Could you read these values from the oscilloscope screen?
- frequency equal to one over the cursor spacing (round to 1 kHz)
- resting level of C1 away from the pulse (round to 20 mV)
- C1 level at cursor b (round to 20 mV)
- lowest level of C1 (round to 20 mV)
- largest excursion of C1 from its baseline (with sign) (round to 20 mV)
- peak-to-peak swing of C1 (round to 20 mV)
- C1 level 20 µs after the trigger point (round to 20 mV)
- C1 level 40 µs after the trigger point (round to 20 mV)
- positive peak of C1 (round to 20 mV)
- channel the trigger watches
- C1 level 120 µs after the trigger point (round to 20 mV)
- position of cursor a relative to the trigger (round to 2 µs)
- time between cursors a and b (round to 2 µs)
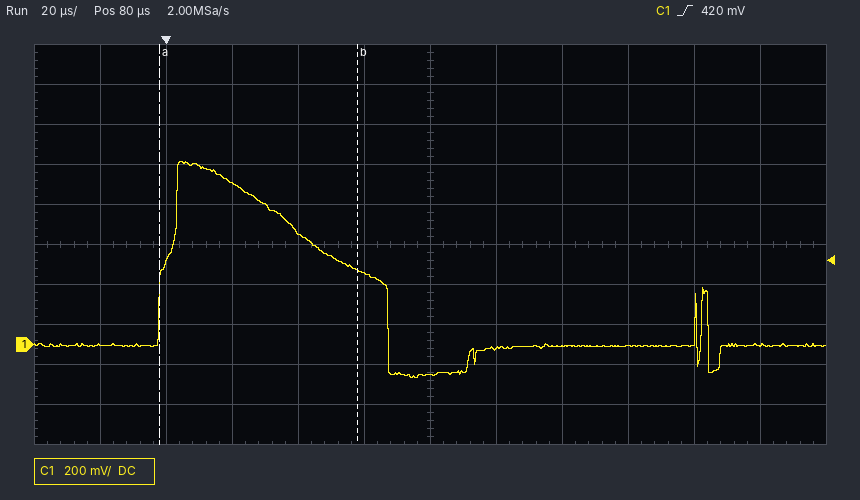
17 kHz
0 mV
380 mV
-160 mV
+920 mV
1.08 V
800 mV
560 mV
920 mV
C1
0 mV
-2 µs
60 µs
